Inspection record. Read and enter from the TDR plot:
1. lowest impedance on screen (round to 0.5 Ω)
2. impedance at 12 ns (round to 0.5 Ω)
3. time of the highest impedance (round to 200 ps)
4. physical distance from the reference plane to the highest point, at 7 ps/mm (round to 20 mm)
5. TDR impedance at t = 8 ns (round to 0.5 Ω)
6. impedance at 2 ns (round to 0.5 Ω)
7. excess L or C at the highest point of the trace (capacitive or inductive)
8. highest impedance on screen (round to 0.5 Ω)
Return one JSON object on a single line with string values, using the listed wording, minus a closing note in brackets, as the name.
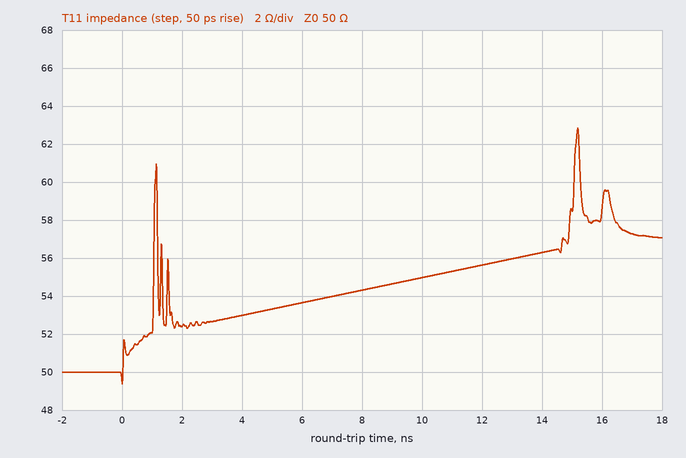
{"lowest impedance on screen": "49.5 Ω", "impedance at 12 ns": "55.5 Ω", "time of the highest impedance": "15.2 ns", "physical distance from the reference plane to the highest point, at 7 ps/mm": "1.08 m", "TDR impedance at t = 8 ns": "54.5 Ω", "impedance at 2 ns": "52.5 Ω", "excess L or C at the highest point of the trace": "inductive", "highest impedance on screen": "63.0 Ω"}
